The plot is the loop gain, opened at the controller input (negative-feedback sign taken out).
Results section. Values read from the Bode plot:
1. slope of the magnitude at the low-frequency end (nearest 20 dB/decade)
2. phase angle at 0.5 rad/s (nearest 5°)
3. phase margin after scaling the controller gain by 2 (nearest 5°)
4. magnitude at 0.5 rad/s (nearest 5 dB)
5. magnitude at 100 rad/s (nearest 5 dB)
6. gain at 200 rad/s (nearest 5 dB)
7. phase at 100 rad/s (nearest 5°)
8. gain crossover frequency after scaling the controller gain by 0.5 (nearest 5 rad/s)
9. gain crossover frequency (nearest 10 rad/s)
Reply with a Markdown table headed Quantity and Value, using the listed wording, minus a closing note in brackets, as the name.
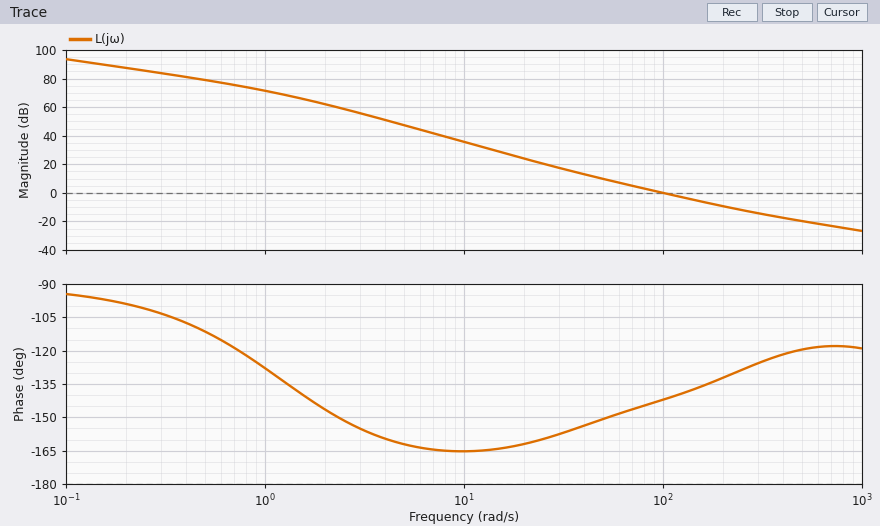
| Quantity | Value |
|---|---|
| slope of the magnitude at the low-frequency end | -20 dB/decade |
| phase angle at 0.5 rad/s | -110° |
| phase margin after scaling the controller gain by 2 | 45° |
| magnitude at 0.5 rad/s | 80 dB |
| magnitude at 100 rad/s | 0 dB |
| gain at 200 rad/s | -10 dB |
| phase at 100 rad/s | -140° |
| gain crossover frequency after scaling the controller gain by 0.5 | 65 rad/s |
| gain crossover frequency | 100 rad/s |
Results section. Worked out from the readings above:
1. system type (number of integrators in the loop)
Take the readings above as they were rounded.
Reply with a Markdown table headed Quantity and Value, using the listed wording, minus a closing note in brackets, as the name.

| Quantity | Value |
|---|---|
| system type | 1 |
